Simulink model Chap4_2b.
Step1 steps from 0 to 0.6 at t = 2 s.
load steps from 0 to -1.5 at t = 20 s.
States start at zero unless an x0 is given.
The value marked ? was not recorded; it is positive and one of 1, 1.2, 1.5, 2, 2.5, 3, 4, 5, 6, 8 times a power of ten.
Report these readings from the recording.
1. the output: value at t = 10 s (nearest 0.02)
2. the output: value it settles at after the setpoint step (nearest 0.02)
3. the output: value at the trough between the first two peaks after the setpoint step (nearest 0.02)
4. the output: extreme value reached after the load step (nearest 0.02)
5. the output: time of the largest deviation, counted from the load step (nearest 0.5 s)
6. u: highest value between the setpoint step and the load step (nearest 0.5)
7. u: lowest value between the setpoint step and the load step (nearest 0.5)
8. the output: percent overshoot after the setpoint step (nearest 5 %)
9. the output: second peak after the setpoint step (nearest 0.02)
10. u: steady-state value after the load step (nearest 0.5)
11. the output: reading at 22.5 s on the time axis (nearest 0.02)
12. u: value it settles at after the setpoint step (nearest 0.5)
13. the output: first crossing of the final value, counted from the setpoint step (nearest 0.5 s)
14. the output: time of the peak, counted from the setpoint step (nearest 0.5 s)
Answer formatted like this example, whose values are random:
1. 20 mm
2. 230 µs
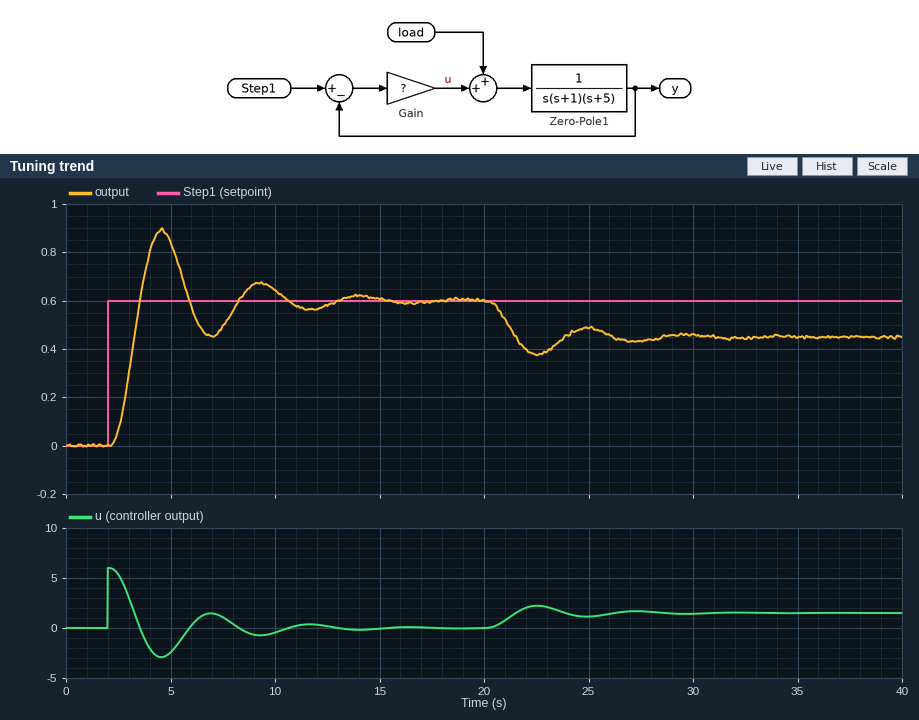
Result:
1. 0.64
2. 0.60
3. 0.46
4. 0.38
5. 2.5 s
6. 6.0
7. -3.0
8. 50 %
9. 0.68
10. 1.5
11. 0.38
12. 0.0
13. 1.5 s
14. 2.5 s
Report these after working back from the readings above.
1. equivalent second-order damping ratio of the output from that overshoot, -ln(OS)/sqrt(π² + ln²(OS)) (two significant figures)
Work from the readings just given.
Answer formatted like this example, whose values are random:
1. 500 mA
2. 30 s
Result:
1. 0.22
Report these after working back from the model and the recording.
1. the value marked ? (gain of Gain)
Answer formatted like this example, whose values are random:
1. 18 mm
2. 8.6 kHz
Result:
1. 10
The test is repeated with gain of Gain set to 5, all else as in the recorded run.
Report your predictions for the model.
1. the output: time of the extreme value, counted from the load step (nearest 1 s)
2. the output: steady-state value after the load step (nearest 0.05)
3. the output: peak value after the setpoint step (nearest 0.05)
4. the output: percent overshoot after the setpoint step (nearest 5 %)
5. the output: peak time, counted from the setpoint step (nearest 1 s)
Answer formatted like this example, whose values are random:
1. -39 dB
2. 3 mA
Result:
1. 4 s
2. 0.30
3. 0.75
4. 25 %
5. 4 s
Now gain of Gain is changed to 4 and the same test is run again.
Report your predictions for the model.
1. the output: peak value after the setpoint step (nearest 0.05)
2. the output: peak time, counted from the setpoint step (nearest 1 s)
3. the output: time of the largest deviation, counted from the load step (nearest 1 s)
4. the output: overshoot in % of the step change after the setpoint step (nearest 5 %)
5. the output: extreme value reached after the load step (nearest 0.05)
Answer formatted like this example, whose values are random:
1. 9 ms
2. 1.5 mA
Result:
1. 0.70
2. 4 s
3. 4 s
4. 20 %
5. 0.15
